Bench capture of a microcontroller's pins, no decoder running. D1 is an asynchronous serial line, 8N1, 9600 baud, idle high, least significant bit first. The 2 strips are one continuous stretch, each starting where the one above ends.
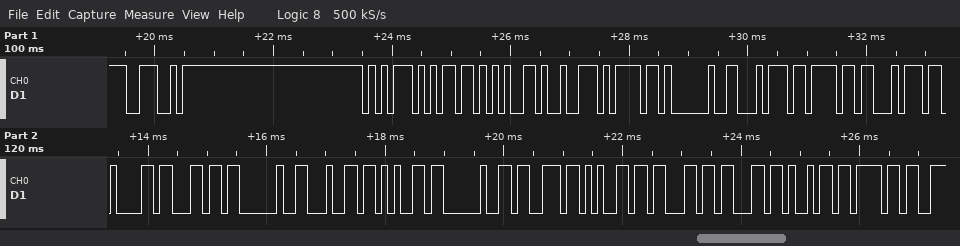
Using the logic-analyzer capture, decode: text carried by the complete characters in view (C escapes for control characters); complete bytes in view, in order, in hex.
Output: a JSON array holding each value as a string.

["\"Numero total de seccio\"", "4E 75 6D 65 72 6F 20 74 6F 74 61 6C 20 64 65 20 73 65 63 63 69 6F"]
